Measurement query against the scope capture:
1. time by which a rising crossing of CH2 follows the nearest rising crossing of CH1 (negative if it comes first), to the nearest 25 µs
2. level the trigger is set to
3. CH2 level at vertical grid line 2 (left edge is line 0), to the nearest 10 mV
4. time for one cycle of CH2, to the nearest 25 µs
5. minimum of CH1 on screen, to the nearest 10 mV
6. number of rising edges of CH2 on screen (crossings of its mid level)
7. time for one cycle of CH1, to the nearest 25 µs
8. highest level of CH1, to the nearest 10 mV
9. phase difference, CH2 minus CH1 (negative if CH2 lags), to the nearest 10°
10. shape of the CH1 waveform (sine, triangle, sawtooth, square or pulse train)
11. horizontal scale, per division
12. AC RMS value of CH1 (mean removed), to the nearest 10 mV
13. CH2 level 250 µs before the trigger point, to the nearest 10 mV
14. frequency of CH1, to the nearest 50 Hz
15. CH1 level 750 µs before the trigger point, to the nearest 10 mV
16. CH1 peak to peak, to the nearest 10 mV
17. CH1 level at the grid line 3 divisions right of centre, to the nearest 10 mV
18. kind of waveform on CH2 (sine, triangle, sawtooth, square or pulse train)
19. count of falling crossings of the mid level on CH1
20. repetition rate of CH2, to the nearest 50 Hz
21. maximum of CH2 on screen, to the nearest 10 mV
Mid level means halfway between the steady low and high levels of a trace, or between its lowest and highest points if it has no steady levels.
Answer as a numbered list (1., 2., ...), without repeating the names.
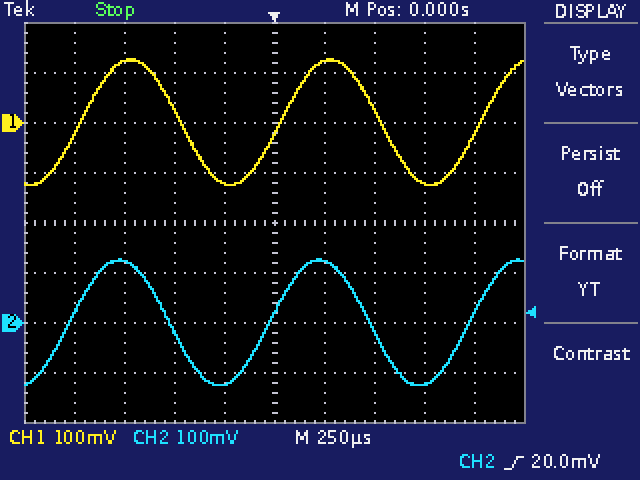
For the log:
1. -50 µs
2. 20.0 mV
3. 120 mV
4. 1.000 ms
5. -120 mV
6. 3
7. 1.000 ms
8. 130 mV
9. +20°
10. sine
11. 250 µs
12. 90 mV
13. -120 mV
14. 1.00 kHz
15. 120 mV
16. 250 mV
17. -120 mV
18. sine
19. 2
20. 1.00 kHz
21. 130 mV
